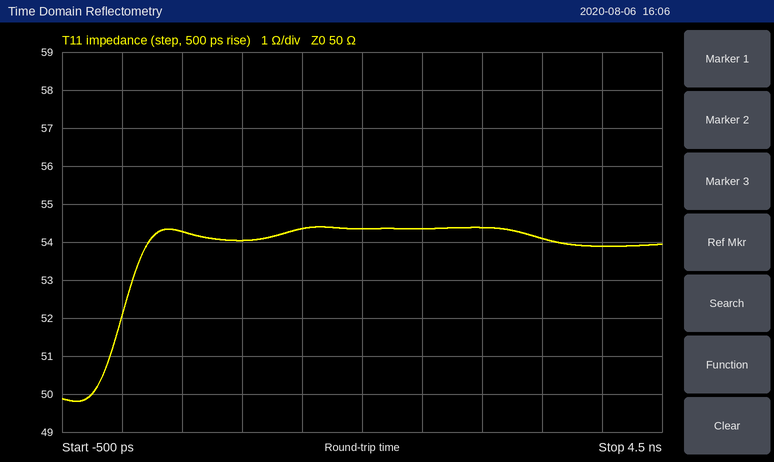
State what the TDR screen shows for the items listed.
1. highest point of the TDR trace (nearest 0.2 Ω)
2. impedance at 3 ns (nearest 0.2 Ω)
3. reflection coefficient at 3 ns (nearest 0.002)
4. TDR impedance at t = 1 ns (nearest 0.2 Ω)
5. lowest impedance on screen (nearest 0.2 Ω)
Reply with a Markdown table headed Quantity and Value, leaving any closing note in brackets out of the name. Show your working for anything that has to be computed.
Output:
| Quantity | Value |
|---|---|
| highest point of the TDR trace | 54.4 Ω |
| impedance at 3 ns | 54.4 Ω |
| reflection coefficient at 3 ns | (54.4 − 50)/(54.4 + 50) ≈ +0.042 |
| TDR impedance at t = 1 ns | 54.0 Ω |
| lowest impedance on screen | 49.8 Ω |
